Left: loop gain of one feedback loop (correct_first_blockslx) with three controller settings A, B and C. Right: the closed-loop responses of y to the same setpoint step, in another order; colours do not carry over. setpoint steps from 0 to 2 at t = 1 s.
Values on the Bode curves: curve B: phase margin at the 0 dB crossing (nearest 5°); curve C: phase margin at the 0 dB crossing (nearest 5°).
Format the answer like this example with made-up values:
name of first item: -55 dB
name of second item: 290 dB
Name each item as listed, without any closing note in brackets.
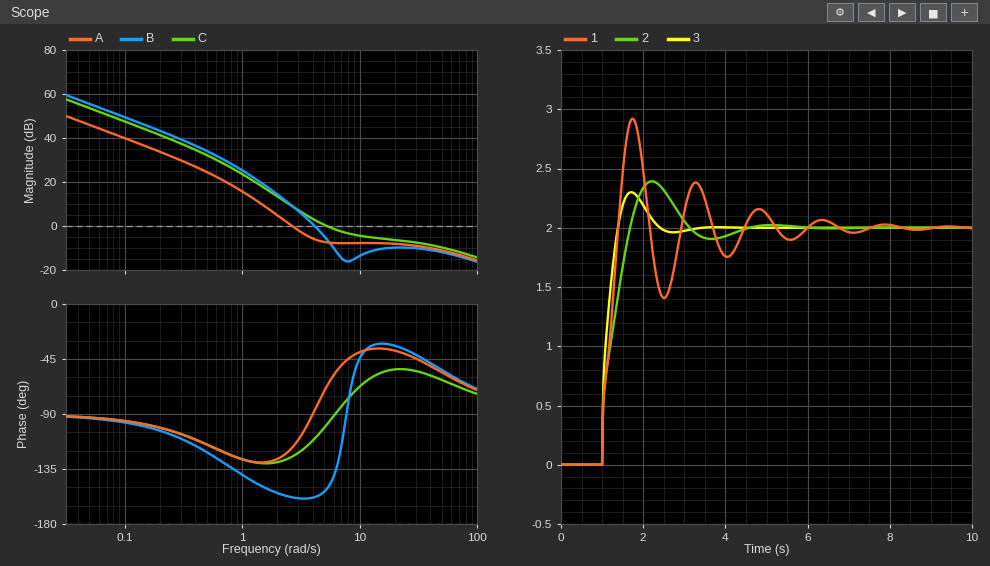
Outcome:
curve B: phase margin at the 0 dB crossing: 20°
curve C: phase margin at the 0 dB crossing: 80°
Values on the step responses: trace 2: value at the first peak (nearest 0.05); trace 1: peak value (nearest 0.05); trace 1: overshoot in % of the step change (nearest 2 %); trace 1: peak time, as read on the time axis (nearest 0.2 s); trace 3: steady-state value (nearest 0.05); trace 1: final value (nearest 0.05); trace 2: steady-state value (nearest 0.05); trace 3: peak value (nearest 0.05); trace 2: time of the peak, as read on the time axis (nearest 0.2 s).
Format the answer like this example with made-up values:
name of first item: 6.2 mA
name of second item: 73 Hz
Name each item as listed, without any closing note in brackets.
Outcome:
trace 2: value at the first peak: 2.40
trace 1: peak value: 2.90
trace 1: overshoot in % of the step change: 46 %
trace 1: peak time, as read on the time axis: 1.8 s
trace 3: steady-state value: 2.00
trace 1: final value: 2.00
trace 2: steady-state value: 2.00
trace 3: peak value: 2.30
trace 2: time of the peak, as read on the time axis: 2.2 s
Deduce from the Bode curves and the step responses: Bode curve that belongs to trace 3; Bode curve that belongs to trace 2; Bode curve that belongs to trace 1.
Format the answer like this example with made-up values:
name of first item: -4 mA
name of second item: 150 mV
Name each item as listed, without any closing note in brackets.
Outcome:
Bode curve that belongs to trace 3: C
Bode curve that belongs to trace 2: A
Bode curve that belongs to trace 1: B
